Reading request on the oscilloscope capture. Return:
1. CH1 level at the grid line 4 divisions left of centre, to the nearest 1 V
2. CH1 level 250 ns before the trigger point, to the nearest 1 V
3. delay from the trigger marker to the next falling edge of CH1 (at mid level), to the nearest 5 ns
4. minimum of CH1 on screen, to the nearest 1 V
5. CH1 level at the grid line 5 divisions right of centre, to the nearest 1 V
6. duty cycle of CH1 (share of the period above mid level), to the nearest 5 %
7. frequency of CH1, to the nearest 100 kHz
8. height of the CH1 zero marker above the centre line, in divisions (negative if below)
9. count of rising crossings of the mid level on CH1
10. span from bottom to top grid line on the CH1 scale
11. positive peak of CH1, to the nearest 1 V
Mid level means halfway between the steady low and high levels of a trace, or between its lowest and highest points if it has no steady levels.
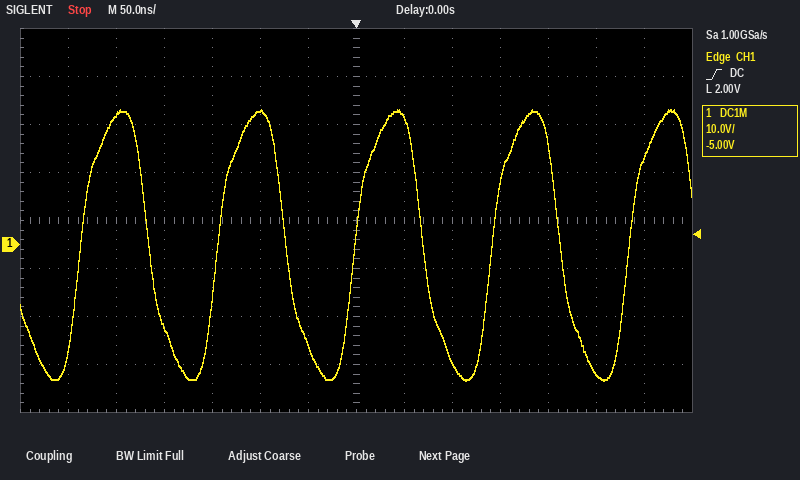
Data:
-17 V
27 V
70 ns
-28 V
-27 V
50 %
7.0 MHz
-0.5 div
5
80 V
28 V
